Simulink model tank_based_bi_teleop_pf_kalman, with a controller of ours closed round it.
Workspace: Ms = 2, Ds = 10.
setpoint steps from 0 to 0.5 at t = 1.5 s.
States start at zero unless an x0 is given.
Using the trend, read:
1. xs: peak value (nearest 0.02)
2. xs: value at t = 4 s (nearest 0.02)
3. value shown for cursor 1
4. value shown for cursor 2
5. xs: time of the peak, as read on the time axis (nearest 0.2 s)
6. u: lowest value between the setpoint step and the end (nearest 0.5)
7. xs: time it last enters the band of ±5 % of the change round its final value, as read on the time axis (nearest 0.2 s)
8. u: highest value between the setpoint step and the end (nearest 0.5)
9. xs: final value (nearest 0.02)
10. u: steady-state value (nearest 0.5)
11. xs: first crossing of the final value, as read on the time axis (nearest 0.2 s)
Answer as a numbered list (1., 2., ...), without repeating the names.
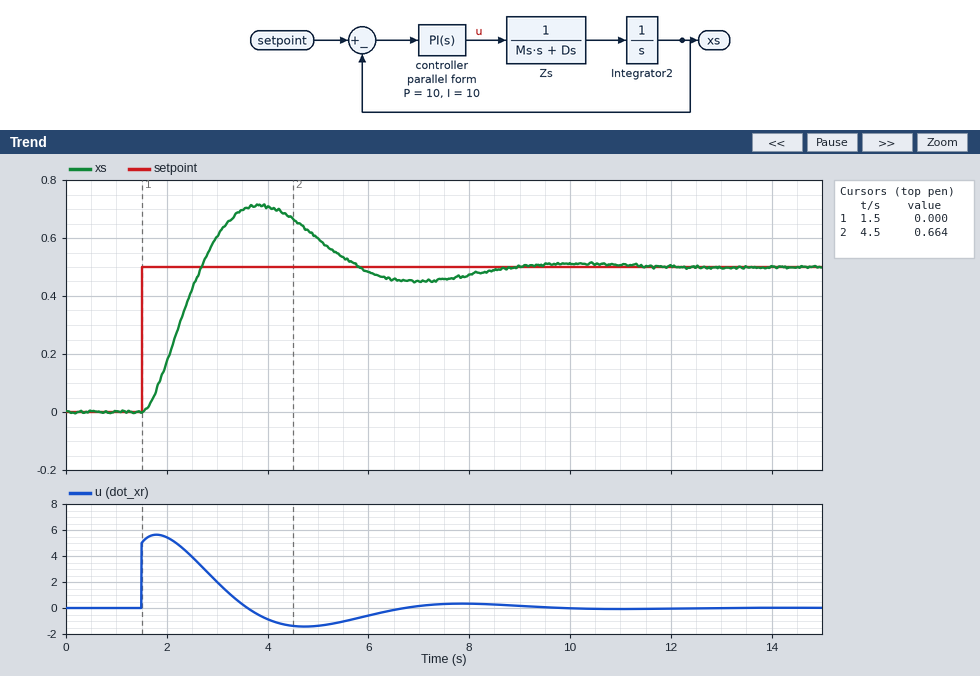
1. 0.72
2. 0.70
3. 0.000
4. 0.664
5. 3.8 s
6. -1.5
7. 8.0 s
8. 5.5
9. 0.50
10. 0.0
11. 2.6 s
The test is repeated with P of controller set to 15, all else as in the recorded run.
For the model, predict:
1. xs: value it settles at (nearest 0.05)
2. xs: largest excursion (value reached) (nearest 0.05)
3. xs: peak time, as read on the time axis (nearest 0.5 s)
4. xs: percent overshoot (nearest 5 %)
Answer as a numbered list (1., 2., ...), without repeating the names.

1. 0.50
2. 0.65
3. 3.5 s
4. 30 %
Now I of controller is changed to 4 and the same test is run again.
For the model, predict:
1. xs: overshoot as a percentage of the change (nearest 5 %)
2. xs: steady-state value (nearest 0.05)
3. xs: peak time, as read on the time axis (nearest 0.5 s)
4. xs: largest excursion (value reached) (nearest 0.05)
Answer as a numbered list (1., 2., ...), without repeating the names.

1. 25 %
2. 0.50
3. 4.5 s
4. 0.60
